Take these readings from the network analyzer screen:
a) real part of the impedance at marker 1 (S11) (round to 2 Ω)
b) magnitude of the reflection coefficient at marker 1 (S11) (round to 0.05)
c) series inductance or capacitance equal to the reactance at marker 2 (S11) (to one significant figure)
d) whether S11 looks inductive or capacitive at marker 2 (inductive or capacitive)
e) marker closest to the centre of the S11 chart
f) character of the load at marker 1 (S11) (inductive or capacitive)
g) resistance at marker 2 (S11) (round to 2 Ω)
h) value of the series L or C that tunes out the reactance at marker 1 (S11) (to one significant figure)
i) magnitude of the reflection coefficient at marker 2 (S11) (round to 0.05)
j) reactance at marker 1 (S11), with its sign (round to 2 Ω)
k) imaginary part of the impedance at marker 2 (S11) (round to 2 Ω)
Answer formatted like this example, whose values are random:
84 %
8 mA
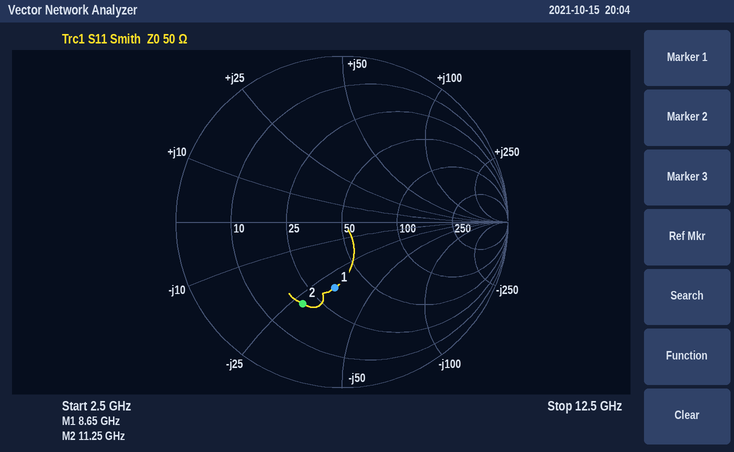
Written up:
34 Ω
0.40
500 fF
capacitive
marker 1
capacitive
20 Ω
600 pH
0.55
-32 Ω
-28 Ω
